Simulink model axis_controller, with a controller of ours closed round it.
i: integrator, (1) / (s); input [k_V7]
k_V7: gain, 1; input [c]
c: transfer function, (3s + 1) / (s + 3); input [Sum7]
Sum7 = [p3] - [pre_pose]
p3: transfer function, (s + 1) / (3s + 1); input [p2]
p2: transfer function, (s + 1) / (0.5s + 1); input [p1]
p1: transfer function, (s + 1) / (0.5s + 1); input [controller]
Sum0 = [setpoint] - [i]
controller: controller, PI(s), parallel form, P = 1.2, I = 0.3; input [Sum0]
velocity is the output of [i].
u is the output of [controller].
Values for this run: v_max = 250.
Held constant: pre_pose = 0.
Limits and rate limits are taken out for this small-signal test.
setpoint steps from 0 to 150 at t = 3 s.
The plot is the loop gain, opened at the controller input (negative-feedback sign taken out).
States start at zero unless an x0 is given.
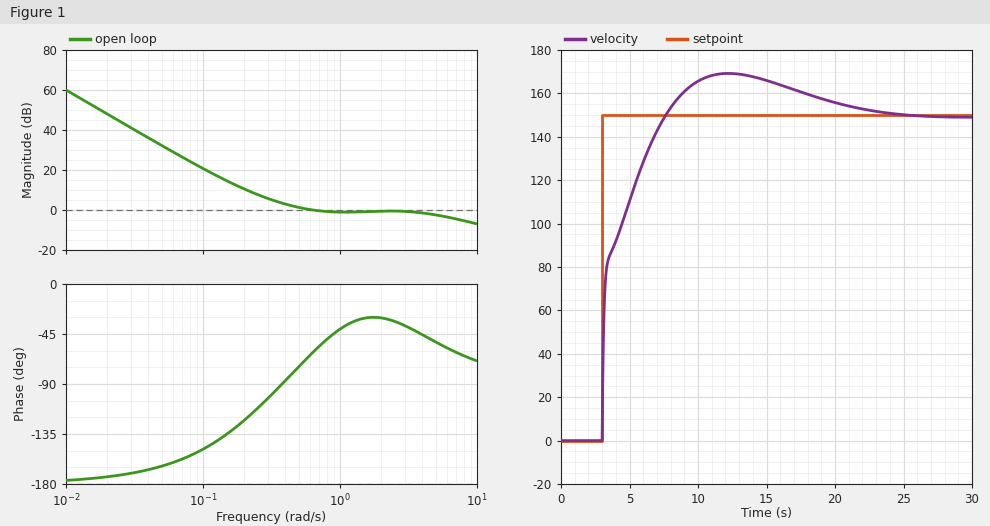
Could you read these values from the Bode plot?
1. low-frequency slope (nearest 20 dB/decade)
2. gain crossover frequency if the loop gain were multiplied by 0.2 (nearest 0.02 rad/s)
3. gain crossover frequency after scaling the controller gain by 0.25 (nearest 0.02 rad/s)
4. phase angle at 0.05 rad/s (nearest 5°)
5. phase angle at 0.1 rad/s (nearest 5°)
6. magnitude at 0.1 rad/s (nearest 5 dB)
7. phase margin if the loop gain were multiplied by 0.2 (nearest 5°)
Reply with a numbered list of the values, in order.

1. -40 dB/decade
2. 0.16 rad/s
3. 0.18 rad/s
4. -165°
5. -150°
6. 20 dB
7. 45°
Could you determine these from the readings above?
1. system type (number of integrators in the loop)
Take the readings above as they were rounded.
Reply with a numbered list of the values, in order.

1. 2
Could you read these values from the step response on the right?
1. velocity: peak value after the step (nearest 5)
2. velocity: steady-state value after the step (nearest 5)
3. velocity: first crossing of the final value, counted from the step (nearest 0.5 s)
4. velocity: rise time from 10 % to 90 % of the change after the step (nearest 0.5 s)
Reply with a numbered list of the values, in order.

1. 170
2. 150
3. 4.5 s
4. 3.5 s
